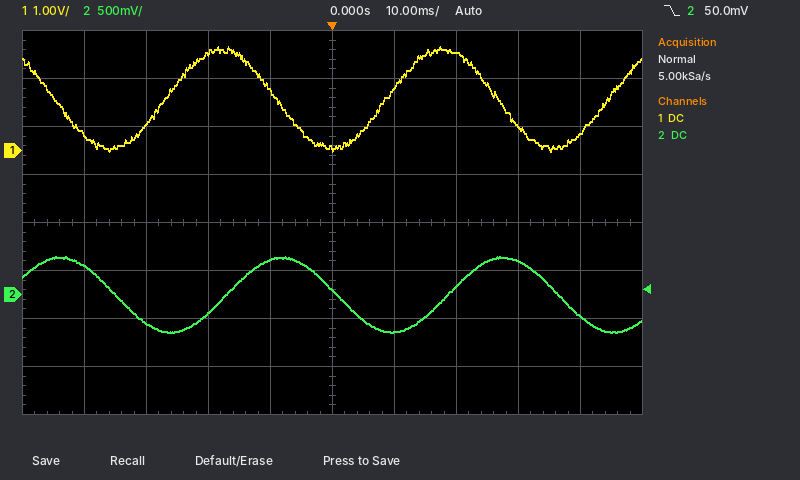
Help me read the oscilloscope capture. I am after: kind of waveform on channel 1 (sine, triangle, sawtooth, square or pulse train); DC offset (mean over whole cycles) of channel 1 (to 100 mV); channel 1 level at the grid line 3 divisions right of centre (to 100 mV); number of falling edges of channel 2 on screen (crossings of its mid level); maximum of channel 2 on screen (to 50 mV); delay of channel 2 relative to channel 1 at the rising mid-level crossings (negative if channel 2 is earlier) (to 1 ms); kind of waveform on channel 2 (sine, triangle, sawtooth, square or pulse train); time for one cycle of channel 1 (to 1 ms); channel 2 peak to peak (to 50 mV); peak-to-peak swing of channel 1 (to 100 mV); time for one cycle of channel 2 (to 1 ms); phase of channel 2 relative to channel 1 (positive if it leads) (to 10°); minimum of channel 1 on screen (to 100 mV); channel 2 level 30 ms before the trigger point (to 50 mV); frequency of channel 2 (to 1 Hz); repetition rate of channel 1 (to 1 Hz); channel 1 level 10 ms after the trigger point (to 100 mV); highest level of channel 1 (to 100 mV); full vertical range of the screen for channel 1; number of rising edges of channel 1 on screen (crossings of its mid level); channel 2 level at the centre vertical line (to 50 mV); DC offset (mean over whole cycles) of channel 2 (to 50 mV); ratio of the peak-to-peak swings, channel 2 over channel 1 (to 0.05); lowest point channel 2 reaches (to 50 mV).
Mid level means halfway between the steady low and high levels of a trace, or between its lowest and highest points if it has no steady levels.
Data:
sine
1.1 V
500 mV
3
400 mV
+10 ms
sine
36 ms
800 mV
2.2 V
36 ms
-100°
0.0 V
-300 mV
28 Hz
28 Hz
1.3 V
2.2 V
8 V
3
50 mV
0 mV
0.35
-400 mV
